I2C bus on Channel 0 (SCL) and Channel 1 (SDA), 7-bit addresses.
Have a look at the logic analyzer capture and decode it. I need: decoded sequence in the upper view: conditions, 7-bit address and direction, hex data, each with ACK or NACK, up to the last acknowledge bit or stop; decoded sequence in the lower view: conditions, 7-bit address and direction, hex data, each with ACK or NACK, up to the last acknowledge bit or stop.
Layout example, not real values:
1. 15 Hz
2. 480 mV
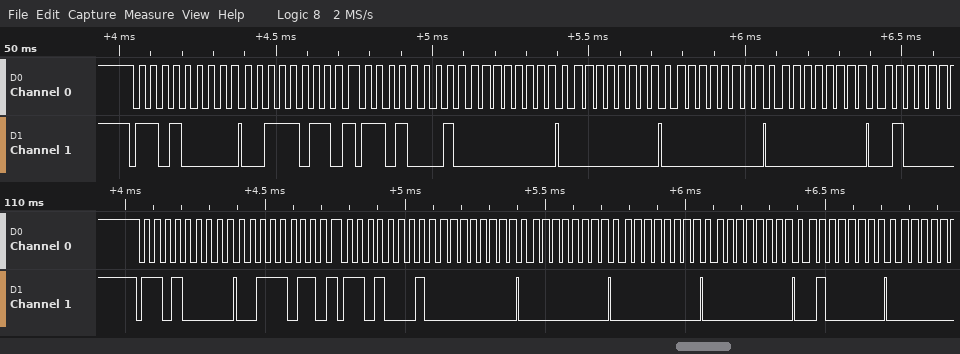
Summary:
1. start, address 68 write ACK, 3B ACK, repeated start, address 68 read ACK, 00 ACK, 00 ACK, 00 ACK, 00 ACK
2. start, address 68 write ACK, 3B ACK, repeated start, address 68 read ACK, 00 ACK, 00 ACK, 00 ACK, 00 ACK, 40 ACK
